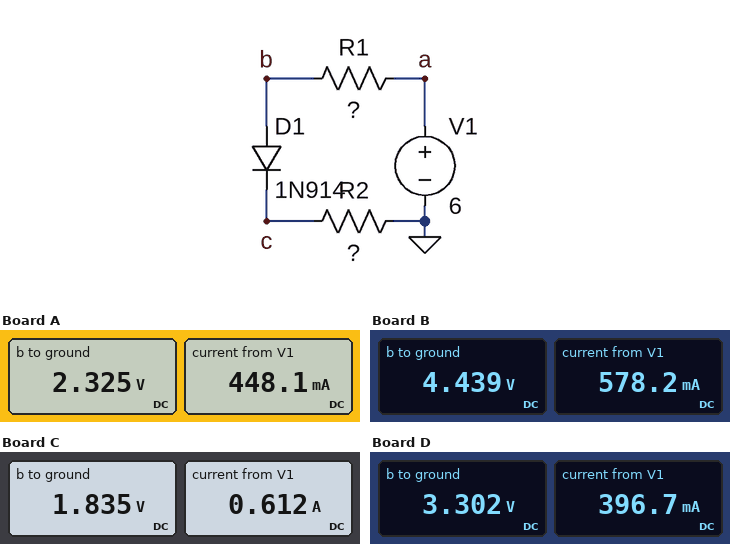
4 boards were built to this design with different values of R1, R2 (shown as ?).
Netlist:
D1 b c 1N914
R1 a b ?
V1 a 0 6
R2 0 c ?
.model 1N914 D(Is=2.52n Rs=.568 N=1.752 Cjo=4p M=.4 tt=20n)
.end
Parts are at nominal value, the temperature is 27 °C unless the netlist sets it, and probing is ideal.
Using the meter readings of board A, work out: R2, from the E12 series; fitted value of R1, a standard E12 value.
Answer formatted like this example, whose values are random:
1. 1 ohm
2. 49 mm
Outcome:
1. 2.7 Ω
2. 8.2 Ω
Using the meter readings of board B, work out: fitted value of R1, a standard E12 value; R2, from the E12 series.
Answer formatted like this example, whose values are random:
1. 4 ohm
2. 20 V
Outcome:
1. 2.7 Ω
2. 5.6 Ω
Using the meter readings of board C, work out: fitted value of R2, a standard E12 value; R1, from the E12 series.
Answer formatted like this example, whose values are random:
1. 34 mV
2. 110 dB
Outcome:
1. 1 Ω
2. 6.8 Ω
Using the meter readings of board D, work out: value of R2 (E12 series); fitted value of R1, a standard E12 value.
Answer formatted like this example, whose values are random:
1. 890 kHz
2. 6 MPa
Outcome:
1. 5.6 Ω
2. 6.8 Ω
